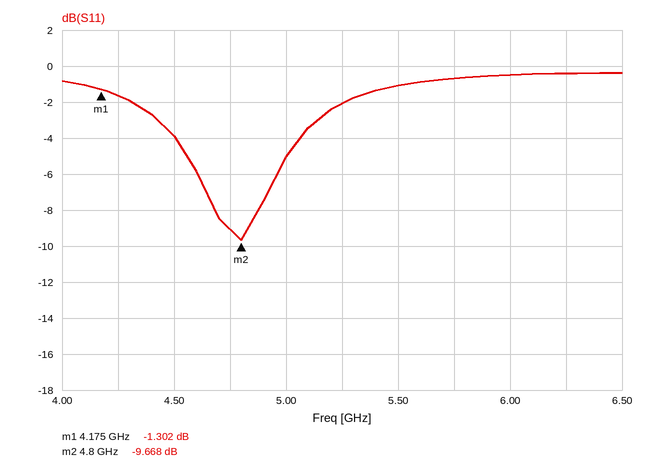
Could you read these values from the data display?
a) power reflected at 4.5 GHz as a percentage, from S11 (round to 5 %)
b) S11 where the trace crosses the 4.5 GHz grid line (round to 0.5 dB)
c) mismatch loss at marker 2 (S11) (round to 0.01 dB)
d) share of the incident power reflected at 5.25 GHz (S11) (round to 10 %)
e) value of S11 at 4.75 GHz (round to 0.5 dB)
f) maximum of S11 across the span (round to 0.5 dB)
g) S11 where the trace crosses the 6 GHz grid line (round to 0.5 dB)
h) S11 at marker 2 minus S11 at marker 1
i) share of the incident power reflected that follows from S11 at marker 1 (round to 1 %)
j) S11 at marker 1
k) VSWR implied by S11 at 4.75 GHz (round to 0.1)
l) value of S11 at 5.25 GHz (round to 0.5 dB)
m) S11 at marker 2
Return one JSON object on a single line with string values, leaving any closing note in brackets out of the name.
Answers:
{"power reflected at 4.5 GHz as a percentage, from S11": "40 %", "S11 where the trace crosses the 4.5 GHz grid line": "-4.0 dB", "mismatch loss at marker 2 (S11)": "0.50 dB", "share of the incident power reflected at 5.25 GHz (S11)": "60 %", "value of S11 at 4.75 GHz": "-9.0 dB", "maximum of S11 across the span": "-0.5 dB", "S11 where the trace crosses the 6 GHz grid line": "-0.5 dB", "S11 at marker 2 minus S11 at marker 1": "-8.366 dB", "share of the incident power reflected that follows from S11 at marker 1": "74 %", "S11 at marker 1": "-1.302 dB", "VSWR implied by S11 at 4.75 GHz": "2.1", "value of S11 at 5.25 GHz": "-2.0 dB", "S11 at marker 2": "-9.668 dB"}
